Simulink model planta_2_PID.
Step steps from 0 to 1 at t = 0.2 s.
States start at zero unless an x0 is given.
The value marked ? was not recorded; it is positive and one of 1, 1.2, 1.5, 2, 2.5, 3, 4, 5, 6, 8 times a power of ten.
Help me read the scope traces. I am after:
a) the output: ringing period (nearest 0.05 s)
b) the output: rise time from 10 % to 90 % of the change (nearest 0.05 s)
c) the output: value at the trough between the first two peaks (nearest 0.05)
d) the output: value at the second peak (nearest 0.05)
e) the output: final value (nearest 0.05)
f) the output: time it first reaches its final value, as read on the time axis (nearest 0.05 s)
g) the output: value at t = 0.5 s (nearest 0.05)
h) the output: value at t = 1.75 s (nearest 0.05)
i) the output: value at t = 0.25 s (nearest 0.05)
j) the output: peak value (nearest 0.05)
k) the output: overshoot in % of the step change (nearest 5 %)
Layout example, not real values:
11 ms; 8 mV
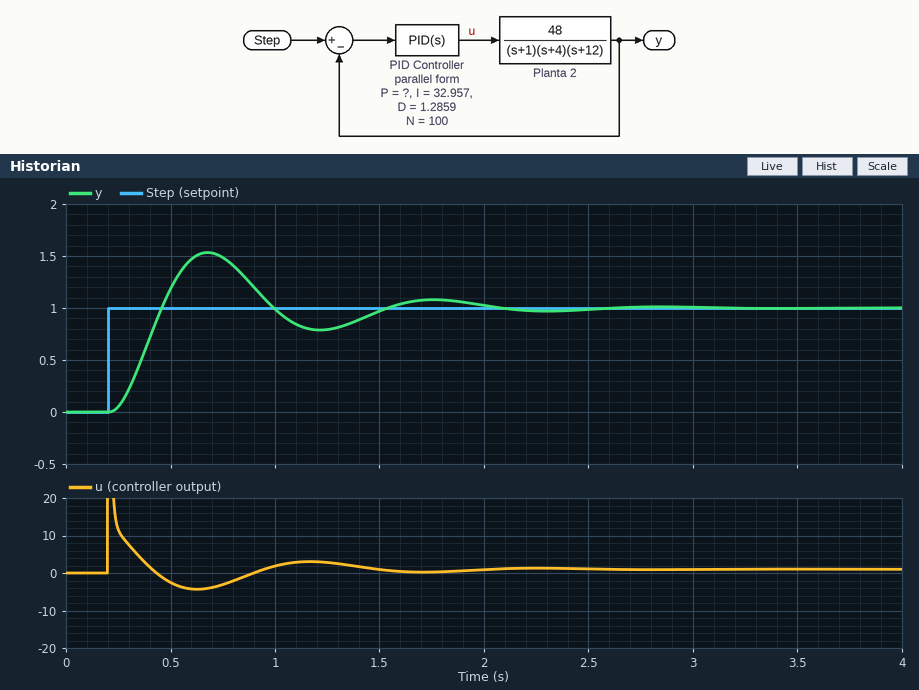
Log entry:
1.10 s; 0.15 s; 0.80; 1.10; 1.00; 0.45 s; 1.20; 1.10; 0.05; 1.55; 55 %
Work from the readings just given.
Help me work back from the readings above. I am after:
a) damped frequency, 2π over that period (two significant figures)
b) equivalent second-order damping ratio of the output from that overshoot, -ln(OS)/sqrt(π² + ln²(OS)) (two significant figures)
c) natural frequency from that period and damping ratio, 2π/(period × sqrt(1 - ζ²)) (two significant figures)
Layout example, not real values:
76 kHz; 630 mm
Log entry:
5.7 rad/s; 0.19; 5.8 rad/s
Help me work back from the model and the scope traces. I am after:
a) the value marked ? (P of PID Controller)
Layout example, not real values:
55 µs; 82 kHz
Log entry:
12
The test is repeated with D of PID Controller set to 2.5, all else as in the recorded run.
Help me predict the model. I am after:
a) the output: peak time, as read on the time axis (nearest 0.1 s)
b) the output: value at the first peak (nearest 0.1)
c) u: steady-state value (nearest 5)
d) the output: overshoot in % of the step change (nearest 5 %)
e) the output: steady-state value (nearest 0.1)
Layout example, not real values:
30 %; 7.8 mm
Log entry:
0.6 s; 1.3; 0; 25 %; 1.0
